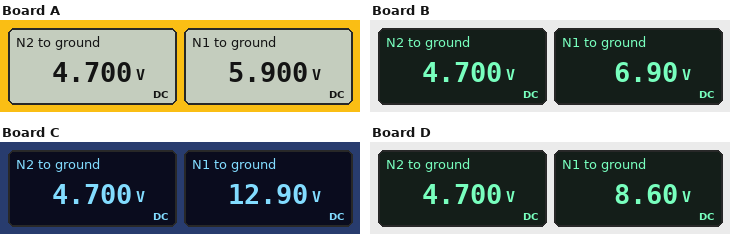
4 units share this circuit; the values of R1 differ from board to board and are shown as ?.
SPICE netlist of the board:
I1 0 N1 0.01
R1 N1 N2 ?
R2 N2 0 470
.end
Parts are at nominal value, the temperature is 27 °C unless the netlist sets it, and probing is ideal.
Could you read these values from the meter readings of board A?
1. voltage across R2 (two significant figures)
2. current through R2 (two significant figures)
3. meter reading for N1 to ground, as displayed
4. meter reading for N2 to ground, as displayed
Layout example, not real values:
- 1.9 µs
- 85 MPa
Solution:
- 4.7 V
- 10 mA
- 5.900 V
- 4.700 V
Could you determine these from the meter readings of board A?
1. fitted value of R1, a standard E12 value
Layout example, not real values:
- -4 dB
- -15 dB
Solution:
- 120 Ω
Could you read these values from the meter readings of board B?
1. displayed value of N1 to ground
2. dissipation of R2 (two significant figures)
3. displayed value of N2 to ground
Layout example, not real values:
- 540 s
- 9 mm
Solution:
- 6.90 V
- 47 mW
- 4.700 V
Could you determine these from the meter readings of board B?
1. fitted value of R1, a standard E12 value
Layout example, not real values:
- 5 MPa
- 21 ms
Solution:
- 220 Ω
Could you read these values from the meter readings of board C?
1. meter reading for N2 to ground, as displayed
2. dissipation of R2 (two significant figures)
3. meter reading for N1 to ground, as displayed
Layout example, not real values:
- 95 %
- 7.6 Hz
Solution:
- 4.700 V
- 47 mW
- 12.90 V
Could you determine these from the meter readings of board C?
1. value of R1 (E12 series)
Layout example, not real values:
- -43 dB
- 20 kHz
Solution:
- 820 Ω
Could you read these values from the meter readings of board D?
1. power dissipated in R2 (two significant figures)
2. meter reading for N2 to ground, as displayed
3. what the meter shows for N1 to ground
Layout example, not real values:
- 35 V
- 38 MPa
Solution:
- 47 mW
- 4.700 V
- 8.60 V
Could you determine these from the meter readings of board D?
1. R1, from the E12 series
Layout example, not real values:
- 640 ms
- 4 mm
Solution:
- 390 Ω
